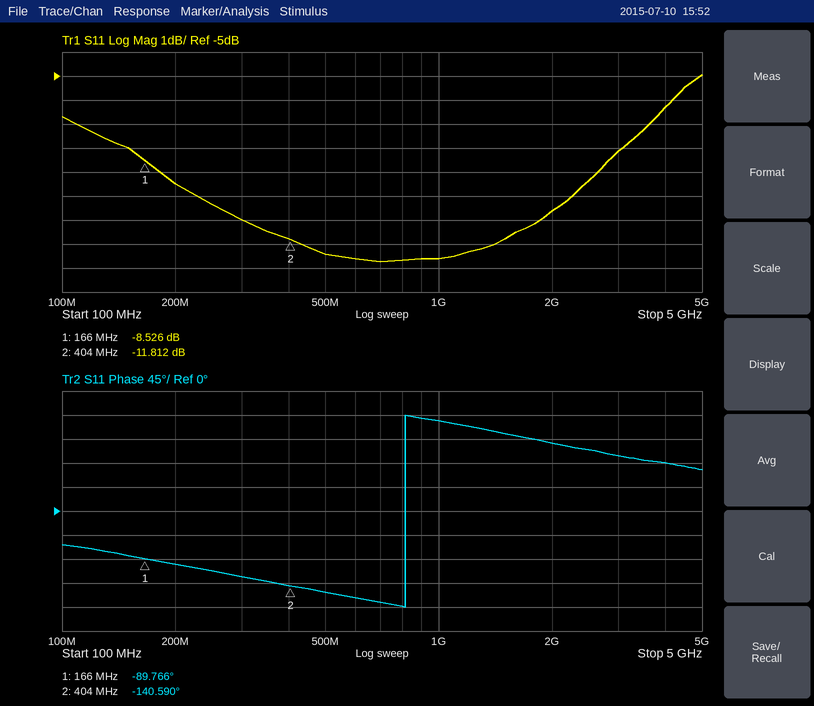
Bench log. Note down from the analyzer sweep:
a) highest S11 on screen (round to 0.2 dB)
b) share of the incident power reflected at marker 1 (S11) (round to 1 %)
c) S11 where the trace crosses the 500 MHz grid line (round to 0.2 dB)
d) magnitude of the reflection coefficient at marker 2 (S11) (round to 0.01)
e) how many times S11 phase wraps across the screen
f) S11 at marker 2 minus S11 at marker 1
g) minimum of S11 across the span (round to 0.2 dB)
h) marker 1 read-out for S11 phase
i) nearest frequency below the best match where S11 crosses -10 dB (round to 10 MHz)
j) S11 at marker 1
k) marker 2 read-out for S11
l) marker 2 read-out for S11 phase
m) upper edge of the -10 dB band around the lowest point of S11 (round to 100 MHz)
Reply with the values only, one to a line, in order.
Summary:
-5.0 dB
14 %
-12.4 dB
0.26
1
-3.286 dB
-12.8 dB
-89.766°
230 MHz
-8.526 dB
-11.812 dB
-140.590°
2.3 GHz
